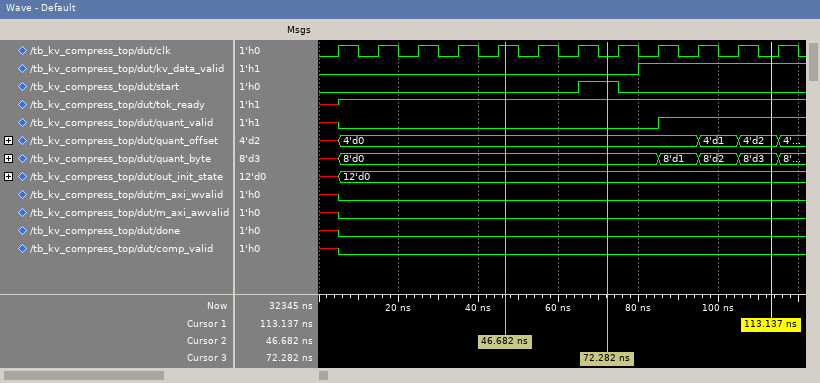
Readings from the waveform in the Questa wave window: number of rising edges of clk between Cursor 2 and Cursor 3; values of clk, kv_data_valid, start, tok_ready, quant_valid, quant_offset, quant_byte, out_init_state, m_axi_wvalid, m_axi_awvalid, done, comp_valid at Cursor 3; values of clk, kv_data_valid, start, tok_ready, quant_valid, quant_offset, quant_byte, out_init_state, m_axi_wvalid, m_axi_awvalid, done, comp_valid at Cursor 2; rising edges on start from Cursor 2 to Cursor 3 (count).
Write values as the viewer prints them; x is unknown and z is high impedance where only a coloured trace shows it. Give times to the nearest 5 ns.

2
clk=0, kv_data_valid=0, start=1, tok_ready=1, quant_valid=0, quant_offset=4'd0, quant_byte=8'd0, out_init_state=12'd0, m_axi_wvalid=0, m_axi_awvalid=0, done=0, comp_valid=0
clk=1, kv_data_valid=0, start=0, tok_ready=1, quant_valid=0, quant_offset=4'd0, quant_byte=8'd0, out_init_state=12'd0, m_axi_wvalid=0, m_axi_awvalid=0, done=0, comp_valid=0
1
